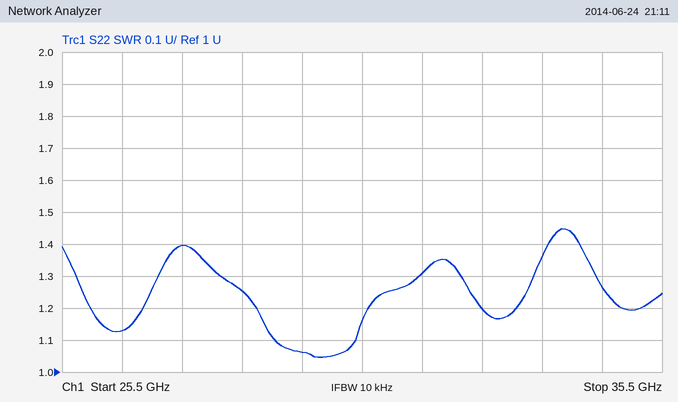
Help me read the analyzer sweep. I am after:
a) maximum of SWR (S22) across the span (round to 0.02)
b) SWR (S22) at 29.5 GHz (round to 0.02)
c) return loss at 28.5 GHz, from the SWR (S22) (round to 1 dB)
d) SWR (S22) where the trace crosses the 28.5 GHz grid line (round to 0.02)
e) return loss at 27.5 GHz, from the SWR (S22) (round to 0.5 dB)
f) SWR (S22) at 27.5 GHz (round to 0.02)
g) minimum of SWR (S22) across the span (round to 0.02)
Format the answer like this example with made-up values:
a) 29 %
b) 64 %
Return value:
a) 1.44
b) 1.06
c) 19 dB
d) 1.26
e) 15.5 dB
f) 1.40
g) 1.04
